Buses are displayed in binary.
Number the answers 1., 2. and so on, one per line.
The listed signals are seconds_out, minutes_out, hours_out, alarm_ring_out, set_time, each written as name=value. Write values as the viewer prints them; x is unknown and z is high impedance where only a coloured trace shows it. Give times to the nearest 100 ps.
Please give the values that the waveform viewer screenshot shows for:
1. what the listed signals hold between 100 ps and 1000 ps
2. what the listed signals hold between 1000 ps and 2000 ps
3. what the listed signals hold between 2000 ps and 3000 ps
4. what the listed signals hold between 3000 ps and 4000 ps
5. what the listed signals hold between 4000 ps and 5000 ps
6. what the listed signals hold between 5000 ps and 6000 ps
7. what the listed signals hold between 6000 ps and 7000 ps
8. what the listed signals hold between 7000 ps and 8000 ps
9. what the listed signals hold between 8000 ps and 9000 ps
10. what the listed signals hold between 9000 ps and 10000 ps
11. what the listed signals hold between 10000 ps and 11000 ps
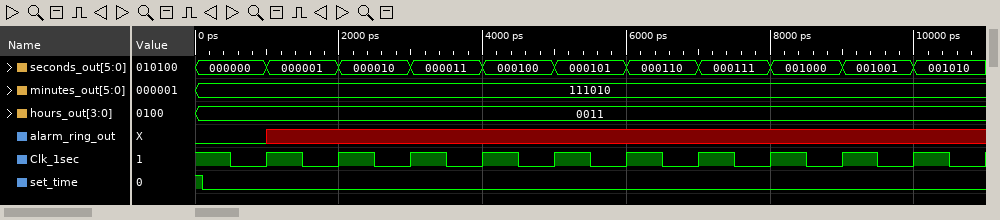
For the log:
1. seconds_out=000000, minutes_out=111010, hours_out=0011, alarm_ring_out=0, set_time=0
2. seconds_out=000001, minutes_out=111010, hours_out=0011, alarm_ring_out=x, set_time=0
3. seconds_out=000010, minutes_out=111010, hours_out=0011, alarm_ring_out=x, set_time=0
4. seconds_out=000011, minutes_out=111010, hours_out=0011, alarm_ring_out=x, set_time=0
5. seconds_out=000100, minutes_out=111010, hours_out=0011, alarm_ring_out=x, set_time=0
6. seconds_out=000101, minutes_out=111010, hours_out=0011, alarm_ring_out=x, set_time=0
7. seconds_out=000110, minutes_out=111010, hours_out=0011, alarm_ring_out=x, set_time=0
8. seconds_out=000111, minutes_out=111010, hours_out=0011, alarm_ring_out=x, set_time=0
9. seconds_out=001000, minutes_out=111010, hours_out=0011, alarm_ring_out=x, set_time=0
10. seconds_out=001001, minutes_out=111010, hours_out=0011, alarm_ring_out=x, set_time=0
11. seconds_out=001010, minutes_out=111010, hours_out=0011, alarm_ring_out=x, set_time=0
